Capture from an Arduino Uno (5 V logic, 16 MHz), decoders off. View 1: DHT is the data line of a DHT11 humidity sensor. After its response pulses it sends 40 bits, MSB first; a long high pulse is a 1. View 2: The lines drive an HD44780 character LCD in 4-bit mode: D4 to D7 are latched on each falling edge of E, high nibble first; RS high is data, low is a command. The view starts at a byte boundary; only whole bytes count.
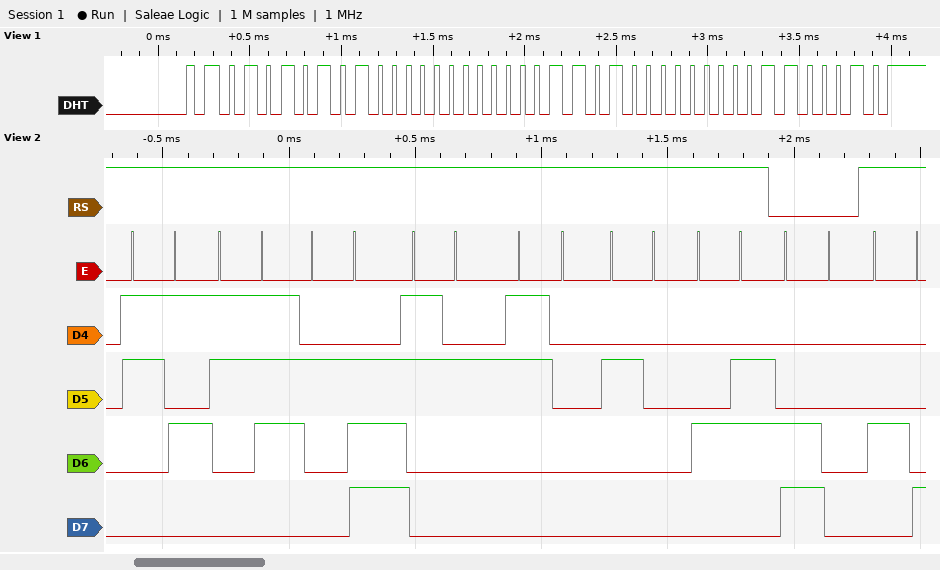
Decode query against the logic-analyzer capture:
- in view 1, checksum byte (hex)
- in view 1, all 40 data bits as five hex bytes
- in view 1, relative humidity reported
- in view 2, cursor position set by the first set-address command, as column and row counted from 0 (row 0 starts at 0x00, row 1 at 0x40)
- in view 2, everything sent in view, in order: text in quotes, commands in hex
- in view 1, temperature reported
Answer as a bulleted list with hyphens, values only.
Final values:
- 0x62
- 55 00 0D 00 62
- 85 %
- column 0, row 1
- "57.20 F" 0xC0 "H"
- 13.0 °C
